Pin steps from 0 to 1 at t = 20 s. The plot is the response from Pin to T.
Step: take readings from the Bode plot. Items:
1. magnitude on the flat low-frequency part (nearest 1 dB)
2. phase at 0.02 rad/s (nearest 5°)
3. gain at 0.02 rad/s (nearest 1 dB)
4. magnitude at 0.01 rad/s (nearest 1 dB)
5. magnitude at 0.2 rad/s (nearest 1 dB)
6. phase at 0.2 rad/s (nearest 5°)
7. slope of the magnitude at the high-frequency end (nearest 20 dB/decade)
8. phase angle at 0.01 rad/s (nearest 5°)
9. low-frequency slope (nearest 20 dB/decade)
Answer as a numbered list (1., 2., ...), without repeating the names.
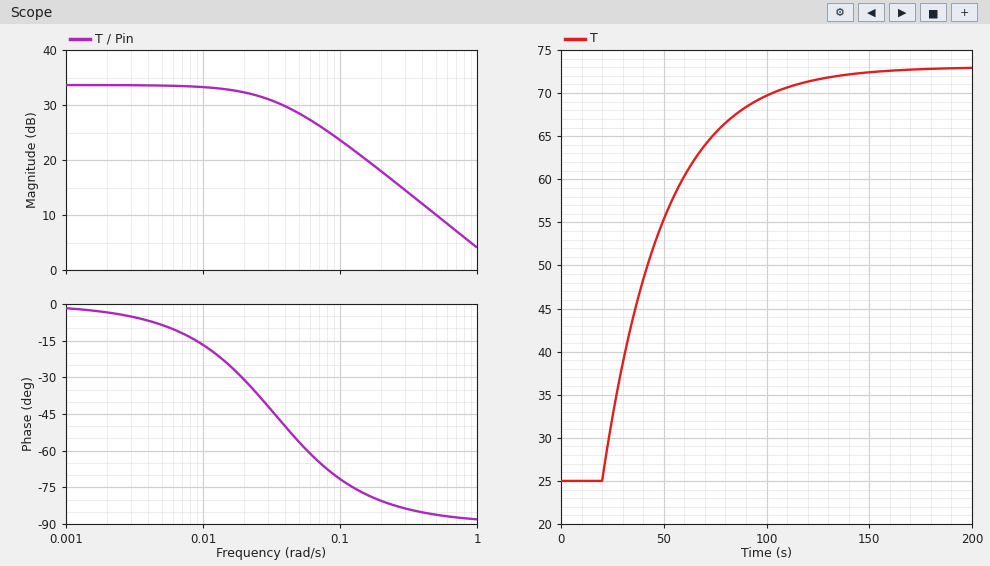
1. 34 dB
2. -30°
3. 32 dB
4. 33 dB
5. 18 dB
6. -80°
7. -20 dB/decade
8. -15°
9. 0 dB/decade
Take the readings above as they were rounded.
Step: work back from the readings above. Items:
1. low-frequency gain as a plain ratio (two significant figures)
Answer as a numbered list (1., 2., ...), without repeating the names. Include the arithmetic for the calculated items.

1. 10^(34 / 20) = 50
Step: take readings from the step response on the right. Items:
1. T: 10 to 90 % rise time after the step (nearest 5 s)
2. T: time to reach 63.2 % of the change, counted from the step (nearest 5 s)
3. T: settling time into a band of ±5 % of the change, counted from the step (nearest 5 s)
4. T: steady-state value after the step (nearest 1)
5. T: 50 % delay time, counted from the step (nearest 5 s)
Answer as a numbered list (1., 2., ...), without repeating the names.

1. 65 s
2. 30 s
3. 90 s
4. 73
5. 20 s
